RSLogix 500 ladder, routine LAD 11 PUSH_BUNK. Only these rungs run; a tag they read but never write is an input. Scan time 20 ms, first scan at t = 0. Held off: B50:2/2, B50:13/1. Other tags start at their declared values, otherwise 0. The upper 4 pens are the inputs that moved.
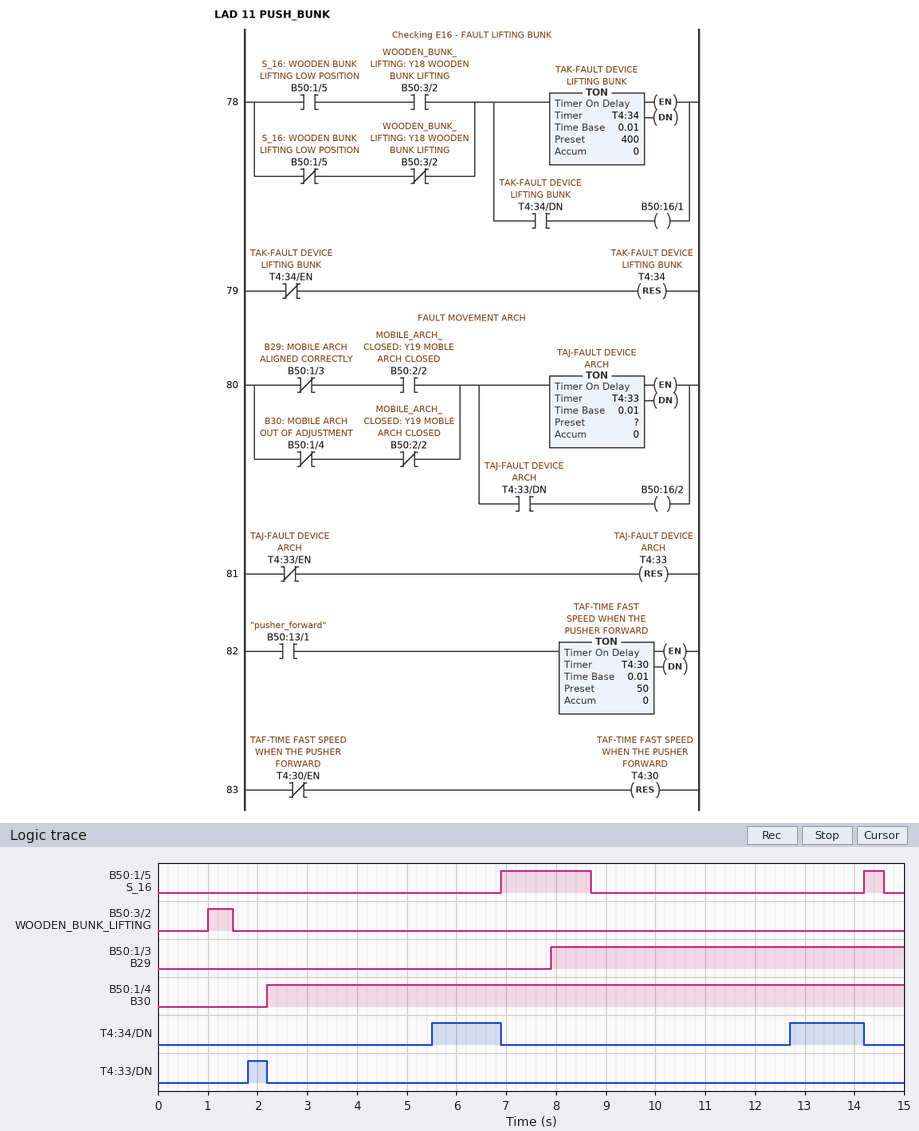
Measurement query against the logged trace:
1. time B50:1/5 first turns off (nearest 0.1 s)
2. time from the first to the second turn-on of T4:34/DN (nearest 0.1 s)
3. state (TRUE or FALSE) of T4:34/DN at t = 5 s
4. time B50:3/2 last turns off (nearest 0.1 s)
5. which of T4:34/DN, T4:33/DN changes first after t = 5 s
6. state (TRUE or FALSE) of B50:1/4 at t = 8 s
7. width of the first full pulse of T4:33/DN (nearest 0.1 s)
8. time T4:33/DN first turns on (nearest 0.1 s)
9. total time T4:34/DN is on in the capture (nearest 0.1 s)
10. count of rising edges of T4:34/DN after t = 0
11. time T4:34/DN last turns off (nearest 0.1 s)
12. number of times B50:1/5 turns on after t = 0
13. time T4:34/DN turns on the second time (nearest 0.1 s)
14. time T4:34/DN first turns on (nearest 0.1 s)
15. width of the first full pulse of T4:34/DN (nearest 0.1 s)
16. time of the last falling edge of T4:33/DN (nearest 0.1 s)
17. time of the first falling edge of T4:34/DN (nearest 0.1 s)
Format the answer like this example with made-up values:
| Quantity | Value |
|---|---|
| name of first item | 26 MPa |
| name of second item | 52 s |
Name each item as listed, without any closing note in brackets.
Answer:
| Quantity | Value |
|---|---|
| time B50:1/5 first turns off | 8.7 s |
| time from the first to the second turn-on of T4:34/DN | 7.2 s |
| state (TRUE or FALSE) of T4:34/DN at t = 5 s | FALSE |
| time B50:3/2 last turns off | 1.5 s |
| which of T4:34/DN, T4:33/DN changes first after t = 5 s | T4:34/DN |
| state (TRUE or FALSE) of B50:1/4 at t = 8 s | TRUE |
| width of the first full pulse of T4:33/DN | 0.4 s |
| time T4:33/DN first turns on | 1.8 s |
| total time T4:34/DN is on in the capture | 2.9 s |
| count of rising edges of T4:34/DN after t = 0 | 2 |
| time T4:34/DN last turns off | 14.2 s |
| number of times B50:1/5 turns on after t = 0 | 2 |
| time T4:34/DN turns on the second time | 12.7 s |
| time T4:34/DN first turns on | 5.5 s |
| width of the first full pulse of T4:34/DN | 1.4 s |
| time of the last falling edge of T4:33/DN | 2.2 s |
| time of the first falling edge of T4:34/DN | 6.9 s |
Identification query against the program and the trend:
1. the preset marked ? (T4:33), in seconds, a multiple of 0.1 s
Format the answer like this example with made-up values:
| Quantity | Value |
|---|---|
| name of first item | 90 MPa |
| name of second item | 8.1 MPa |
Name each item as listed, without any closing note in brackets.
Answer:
| Quantity | Value |
|---|---|
| the preset marked ? (T4:33), in seconds, a multiple of 0.1 s | 1.8 s |
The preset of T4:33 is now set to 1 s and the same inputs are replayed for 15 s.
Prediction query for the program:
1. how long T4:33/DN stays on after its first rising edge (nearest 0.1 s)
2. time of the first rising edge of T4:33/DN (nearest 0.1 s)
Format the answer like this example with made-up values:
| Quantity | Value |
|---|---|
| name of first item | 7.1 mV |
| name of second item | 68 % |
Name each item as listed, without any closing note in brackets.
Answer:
| Quantity | Value |
|---|---|
| how long T4:33/DN stays on after its first rising edge | 1.2 s |
| time of the first rising edge of T4:33/DN | 1.0 s |
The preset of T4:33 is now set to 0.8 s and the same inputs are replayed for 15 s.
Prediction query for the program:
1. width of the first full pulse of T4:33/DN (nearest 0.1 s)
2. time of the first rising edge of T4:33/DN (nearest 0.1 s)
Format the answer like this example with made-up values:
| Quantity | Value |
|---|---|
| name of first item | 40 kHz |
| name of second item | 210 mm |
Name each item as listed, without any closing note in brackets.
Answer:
| Quantity | Value |
|---|---|
| width of the first full pulse of T4:33/DN | 1.4 s |
| time of the first rising edge of T4:33/DN | 0.8 s |
